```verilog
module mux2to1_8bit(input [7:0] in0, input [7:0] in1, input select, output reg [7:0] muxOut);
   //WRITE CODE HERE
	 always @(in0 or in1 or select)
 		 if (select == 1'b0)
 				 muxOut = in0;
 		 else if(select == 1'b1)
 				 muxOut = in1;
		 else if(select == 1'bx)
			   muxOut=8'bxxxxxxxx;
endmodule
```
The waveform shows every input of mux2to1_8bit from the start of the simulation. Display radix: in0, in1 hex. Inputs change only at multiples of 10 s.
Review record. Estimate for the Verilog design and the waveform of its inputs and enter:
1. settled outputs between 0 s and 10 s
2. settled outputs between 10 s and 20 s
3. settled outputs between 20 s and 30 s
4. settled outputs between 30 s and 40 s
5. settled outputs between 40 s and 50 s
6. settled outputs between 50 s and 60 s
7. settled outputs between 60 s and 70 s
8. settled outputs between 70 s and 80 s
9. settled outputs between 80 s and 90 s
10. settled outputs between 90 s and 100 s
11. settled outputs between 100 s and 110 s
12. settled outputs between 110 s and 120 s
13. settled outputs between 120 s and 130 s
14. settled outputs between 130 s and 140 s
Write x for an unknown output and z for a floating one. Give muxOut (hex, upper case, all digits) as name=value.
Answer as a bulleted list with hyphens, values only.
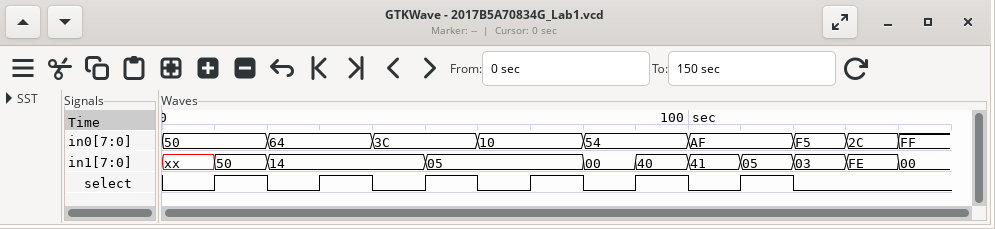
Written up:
- muxOut=50
- muxOut=50
- muxOut=64
- muxOut=14
- muxOut=3C
- muxOut=05
- muxOut=10
- muxOut=05
- muxOut=54
- muxOut=40
- muxOut=AF
- muxOut=05
- muxOut=F5
- muxOut=2C
